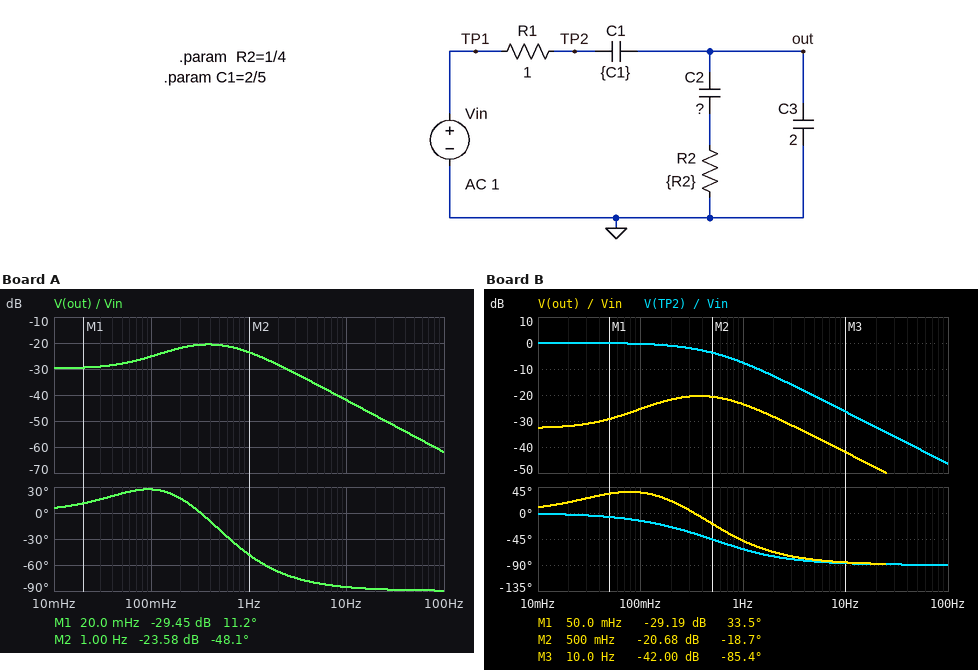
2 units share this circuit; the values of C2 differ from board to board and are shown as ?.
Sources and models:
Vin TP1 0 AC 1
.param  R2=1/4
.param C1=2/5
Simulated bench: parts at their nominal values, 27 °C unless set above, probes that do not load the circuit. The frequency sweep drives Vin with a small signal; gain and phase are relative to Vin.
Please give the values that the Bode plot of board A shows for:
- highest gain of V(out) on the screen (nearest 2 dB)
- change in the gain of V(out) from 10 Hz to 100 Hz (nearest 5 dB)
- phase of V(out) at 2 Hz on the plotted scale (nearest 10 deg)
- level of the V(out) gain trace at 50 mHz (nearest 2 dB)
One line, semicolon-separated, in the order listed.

-20 dB; -20 dB; -70 deg; -28 dB
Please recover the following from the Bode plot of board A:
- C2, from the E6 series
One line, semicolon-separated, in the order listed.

10 F
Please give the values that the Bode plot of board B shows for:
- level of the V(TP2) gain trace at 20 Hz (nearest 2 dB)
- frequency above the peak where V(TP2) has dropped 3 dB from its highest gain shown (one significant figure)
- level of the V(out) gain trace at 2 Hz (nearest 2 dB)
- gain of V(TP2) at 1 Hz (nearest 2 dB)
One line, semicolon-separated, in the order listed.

-32 dB; 400 mHz; -28 dB; -8 dB
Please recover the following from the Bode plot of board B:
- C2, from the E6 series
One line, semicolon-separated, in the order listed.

15 F
